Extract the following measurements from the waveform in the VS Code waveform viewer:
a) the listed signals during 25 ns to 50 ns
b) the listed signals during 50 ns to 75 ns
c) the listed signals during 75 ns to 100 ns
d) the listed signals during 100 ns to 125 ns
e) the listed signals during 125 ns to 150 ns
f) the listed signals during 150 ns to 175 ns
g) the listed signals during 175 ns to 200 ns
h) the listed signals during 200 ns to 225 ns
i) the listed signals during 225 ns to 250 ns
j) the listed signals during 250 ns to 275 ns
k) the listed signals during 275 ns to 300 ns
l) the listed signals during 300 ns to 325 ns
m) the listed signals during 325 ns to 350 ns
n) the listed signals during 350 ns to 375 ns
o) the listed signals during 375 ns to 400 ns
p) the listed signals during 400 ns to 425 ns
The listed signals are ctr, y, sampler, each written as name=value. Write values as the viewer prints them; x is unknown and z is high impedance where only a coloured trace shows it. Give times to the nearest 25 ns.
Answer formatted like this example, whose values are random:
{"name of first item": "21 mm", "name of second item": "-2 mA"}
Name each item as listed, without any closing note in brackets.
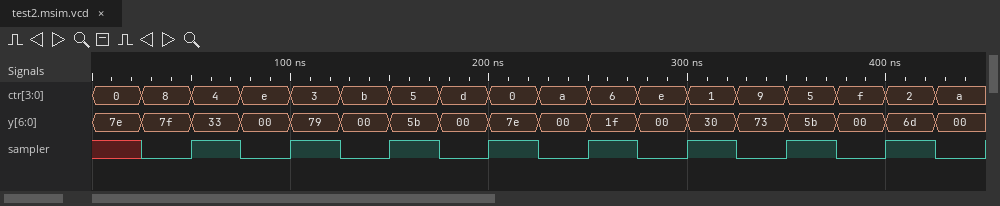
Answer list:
{"the listed signals during 25 ns to 50 ns": "ctr=8, y=7f, sampler=0", "the listed signals during 50 ns to 75 ns": "ctr=4, y=33, sampler=1", "the listed signals during 75 ns to 100 ns": "ctr=e, y=00, sampler=0", "the listed signals during 100 ns to 125 ns": "ctr=3, y=79, sampler=1", "the listed signals during 125 ns to 150 ns": "ctr=b, y=00, sampler=0", "the listed signals during 150 ns to 175 ns": "ctr=5, y=5b, sampler=1", "the listed signals during 175 ns to 200 ns": "ctr=d, y=00, sampler=0", "the listed signals during 200 ns to 225 ns": "ctr=0, y=7e, sampler=1", "the listed signals during 225 ns to 250 ns": "ctr=a, y=00, sampler=0", "the listed signals during 250 ns to 275 ns": "ctr=6, y=1f, sampler=1", "the listed signals during 275 ns to 300 ns": "ctr=e, y=00, sampler=0", "the listed signals during 300 ns to 325 ns": "ctr=1, y=30, sampler=1", "the listed signals during 325 ns to 350 ns": "ctr=9, y=73, sampler=0", "the listed signals during 350 ns to 375 ns": "ctr=5, y=5b, sampler=1", "the listed signals during 375 ns to 400 ns": "ctr=f, y=00, sampler=0", "the listed signals during 400 ns to 425 ns": "ctr=2, y=6d, sampler=1"}
